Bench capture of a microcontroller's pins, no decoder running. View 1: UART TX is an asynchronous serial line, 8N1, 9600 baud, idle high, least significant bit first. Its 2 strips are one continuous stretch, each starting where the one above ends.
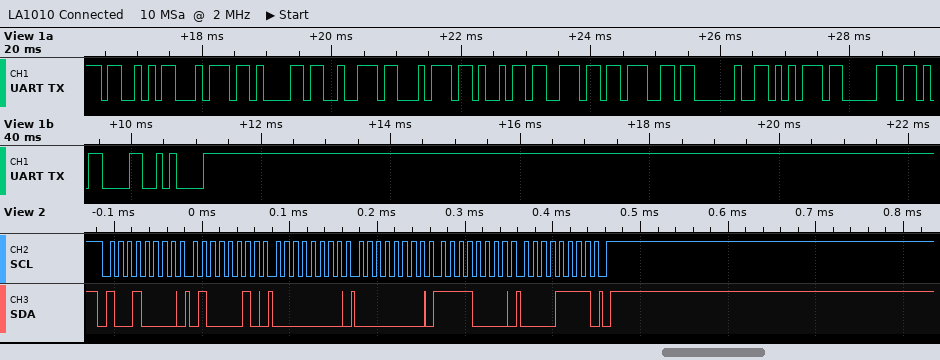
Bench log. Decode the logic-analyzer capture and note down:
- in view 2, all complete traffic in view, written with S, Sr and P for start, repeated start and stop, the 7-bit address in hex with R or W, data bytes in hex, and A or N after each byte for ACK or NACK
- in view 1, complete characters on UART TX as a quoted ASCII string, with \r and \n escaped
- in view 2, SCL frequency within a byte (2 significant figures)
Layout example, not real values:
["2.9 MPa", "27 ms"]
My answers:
["S 48W A 42 A 00 A 00 A F0 A 0F A P", "\"Starting up\\r\\n\"", "100 kHz"]
